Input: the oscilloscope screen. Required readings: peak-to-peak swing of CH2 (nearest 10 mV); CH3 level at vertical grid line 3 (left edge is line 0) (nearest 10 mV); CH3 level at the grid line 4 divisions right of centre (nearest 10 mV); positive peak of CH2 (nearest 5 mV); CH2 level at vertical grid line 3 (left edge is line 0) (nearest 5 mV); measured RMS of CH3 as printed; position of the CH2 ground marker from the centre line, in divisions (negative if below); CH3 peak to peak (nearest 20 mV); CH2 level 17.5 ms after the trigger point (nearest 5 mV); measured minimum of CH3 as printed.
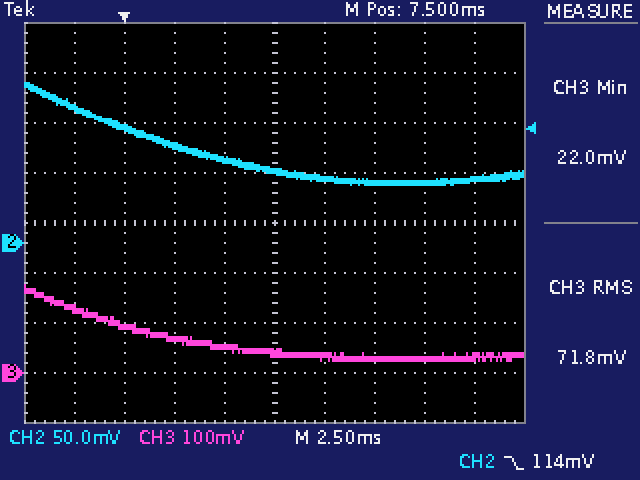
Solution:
100 mV
70 mV
30 mV
160 mV
95 mV
71.8 mV
-0.4 div
160 mV
65 mV
22.0 mV
